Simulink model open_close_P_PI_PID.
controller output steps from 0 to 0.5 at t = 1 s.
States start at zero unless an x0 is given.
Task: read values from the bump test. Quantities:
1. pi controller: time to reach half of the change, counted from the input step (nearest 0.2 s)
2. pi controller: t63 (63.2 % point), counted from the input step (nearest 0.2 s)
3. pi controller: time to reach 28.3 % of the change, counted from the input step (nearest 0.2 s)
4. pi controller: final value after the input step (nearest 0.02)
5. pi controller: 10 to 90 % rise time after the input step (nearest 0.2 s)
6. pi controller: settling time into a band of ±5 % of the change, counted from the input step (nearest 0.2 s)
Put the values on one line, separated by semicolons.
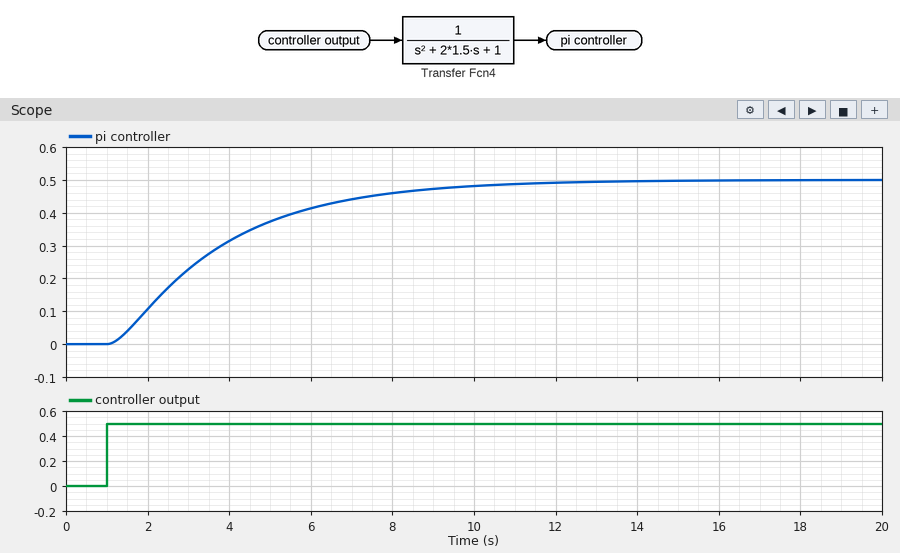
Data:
2.2 s; 3.0 s; 1.2 s; 0.50; 5.8 s; 8.2 s
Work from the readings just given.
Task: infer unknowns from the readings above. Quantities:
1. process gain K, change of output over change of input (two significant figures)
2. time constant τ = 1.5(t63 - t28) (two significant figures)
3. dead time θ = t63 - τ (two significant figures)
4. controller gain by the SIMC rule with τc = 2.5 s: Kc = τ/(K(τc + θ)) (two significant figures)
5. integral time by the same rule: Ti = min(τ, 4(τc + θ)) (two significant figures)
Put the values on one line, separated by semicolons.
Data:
1.0; 2.7 s; 0.30 s; 0.96; 2.7 s
